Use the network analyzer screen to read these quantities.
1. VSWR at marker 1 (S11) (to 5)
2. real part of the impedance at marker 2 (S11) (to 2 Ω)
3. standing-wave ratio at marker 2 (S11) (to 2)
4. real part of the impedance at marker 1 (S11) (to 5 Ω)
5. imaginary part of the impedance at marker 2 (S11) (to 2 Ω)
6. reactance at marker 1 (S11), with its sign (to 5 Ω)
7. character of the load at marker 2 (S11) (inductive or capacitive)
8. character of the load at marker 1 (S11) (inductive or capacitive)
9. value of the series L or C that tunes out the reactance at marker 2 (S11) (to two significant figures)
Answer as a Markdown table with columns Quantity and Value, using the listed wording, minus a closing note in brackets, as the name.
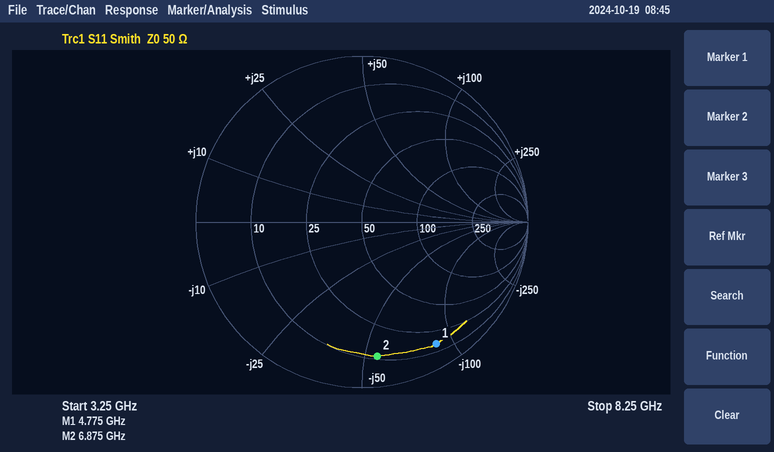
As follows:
| Quantity | Value |
|---|---|
| VSWR at marker 1 (S11) | 15 |
| real part of the impedance at marker 2 (S11) | 12 Ω |
| standing-wave ratio at marker 2 (S11) | 10 |
| real part of the impedance at marker 1 (S11) | 15 Ω |
| imaginary part of the impedance at marker 2 (S11) | -54 Ω |
| reactance at marker 1 (S11), with its sign | -85 Ω |
| character of the load at marker 2 (S11) | capacitive |
| character of the load at marker 1 (S11) | capacitive |
| value of the series L or C that tunes out the reactance at marker 2 (S11) | 1.3 nH |
